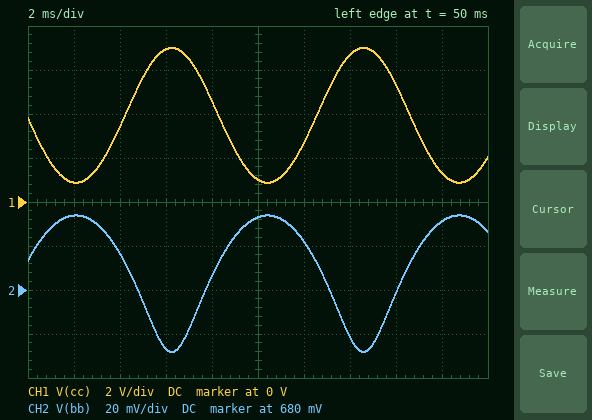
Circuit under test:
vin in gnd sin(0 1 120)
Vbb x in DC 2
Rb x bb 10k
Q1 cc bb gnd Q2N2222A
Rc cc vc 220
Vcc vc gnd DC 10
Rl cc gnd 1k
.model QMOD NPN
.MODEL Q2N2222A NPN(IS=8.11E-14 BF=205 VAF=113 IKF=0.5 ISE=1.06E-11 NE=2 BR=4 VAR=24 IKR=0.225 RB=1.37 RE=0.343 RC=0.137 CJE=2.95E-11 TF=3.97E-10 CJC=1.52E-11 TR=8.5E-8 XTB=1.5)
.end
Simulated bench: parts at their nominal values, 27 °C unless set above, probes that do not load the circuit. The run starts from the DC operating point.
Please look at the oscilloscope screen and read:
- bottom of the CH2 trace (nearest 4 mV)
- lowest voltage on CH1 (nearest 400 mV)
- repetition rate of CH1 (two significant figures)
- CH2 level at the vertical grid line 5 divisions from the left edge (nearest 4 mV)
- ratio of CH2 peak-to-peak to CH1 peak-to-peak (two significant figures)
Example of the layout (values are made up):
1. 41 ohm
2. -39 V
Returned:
1. 652 mV
2. 800 mV
3. 120 Hz
4. 712 mV
5. 0.010
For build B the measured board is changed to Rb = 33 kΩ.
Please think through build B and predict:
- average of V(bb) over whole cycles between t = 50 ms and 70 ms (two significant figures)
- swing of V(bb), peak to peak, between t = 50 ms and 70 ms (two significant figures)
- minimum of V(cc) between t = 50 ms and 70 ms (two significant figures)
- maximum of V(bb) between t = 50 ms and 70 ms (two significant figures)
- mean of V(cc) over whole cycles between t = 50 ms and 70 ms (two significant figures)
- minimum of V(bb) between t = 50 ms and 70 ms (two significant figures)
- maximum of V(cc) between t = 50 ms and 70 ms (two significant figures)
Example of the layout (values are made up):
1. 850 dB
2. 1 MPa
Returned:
1. 650 mV
2. 53 mV
3. 5.8 V
4. 670 mV
5. 6.8 V
6. 620 mV
7. 7.8 V
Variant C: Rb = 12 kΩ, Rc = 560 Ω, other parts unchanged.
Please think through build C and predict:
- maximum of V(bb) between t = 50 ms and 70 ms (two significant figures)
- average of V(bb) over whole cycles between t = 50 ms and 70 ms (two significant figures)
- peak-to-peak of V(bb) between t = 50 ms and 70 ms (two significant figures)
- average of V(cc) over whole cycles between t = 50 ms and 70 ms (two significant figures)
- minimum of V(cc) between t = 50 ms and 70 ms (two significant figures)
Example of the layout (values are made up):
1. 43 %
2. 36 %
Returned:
1. 680 mV
2. 670 mV
3. 37 mV
4. 1.4 V
5. 110 mV
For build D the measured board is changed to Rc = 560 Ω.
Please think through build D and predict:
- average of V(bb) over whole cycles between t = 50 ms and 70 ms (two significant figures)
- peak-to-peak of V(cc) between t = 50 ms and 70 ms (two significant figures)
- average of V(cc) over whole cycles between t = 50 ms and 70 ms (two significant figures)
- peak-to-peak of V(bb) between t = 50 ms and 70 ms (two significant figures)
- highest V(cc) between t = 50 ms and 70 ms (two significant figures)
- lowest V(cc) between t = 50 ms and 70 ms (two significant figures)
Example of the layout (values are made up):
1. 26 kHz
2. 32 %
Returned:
1. 680 mV
2. 4.0 V
3. 1.1 V
4. 33 mV
5. 4.1 V
6. 100 mV
